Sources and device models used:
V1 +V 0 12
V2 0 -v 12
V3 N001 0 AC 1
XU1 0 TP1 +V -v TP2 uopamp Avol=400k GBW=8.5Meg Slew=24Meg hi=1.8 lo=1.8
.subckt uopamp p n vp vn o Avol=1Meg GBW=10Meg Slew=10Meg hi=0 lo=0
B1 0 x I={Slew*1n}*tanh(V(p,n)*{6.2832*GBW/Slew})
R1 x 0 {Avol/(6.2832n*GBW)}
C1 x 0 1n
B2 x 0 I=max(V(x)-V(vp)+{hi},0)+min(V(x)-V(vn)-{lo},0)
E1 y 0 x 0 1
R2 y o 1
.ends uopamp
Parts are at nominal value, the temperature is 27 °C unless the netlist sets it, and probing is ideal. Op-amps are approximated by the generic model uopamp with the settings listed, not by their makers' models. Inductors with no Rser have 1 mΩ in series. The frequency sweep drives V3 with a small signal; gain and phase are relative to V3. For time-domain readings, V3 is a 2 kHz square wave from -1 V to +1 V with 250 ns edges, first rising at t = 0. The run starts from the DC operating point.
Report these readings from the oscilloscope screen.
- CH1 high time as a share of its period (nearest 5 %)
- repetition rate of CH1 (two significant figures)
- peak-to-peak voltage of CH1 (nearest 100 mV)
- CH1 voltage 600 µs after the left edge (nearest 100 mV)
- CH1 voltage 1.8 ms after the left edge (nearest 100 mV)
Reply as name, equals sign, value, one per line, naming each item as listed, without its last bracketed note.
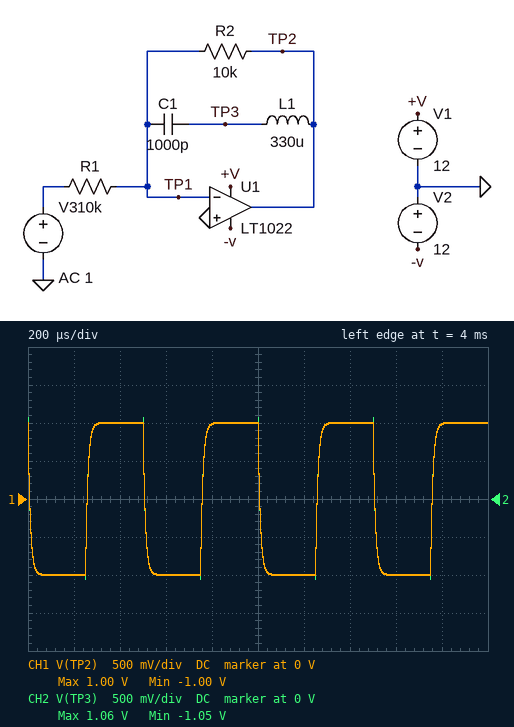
CH1 high time as a share of its period = 50 %
repetition rate of CH1 = 2.0 kHz
peak-to-peak voltage of CH1 = 2.0 V
CH1 voltage 600 µs after the left edge = -1.0 V
CH1 voltage 1.8 ms after the left edge = 1.0 V
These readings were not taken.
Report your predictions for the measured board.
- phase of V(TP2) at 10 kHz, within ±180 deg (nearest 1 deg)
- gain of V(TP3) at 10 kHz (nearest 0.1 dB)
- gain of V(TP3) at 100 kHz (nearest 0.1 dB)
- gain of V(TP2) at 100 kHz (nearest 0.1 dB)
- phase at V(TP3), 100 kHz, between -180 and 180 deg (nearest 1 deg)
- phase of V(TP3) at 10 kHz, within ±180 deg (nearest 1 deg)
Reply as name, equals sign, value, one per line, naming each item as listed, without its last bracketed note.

phase of V(TP2) at 10 kHz, within ±180 deg = 148 deg
gain of V(TP3) at 10 kHz = -1.4 dB
gain of V(TP3) at 100 kHz = -16.1 dB
gain of V(TP2) at 100 kHz = -17.3 dB
phase at V(TP3), 100 kHz, between -180 and 180 deg = 97 deg
phase of V(TP3) at 10 kHz, within ±180 deg = 148 deg
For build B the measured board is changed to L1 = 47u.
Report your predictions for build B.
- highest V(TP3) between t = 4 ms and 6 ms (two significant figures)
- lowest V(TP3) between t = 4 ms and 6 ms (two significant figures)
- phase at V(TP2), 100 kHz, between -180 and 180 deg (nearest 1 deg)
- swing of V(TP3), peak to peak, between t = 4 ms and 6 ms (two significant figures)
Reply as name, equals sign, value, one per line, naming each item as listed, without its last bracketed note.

highest V(TP3) between t = 4 ms and 6 ms = 1.0 V
lowest V(TP3) between t = 4 ms and 6 ms = -1.0 V
phase at V(TP2), 100 kHz, between -180 and 180 deg = 98 deg
swing of V(TP3), peak to peak, between t = 4 ms and 6 ms = 2.0 V
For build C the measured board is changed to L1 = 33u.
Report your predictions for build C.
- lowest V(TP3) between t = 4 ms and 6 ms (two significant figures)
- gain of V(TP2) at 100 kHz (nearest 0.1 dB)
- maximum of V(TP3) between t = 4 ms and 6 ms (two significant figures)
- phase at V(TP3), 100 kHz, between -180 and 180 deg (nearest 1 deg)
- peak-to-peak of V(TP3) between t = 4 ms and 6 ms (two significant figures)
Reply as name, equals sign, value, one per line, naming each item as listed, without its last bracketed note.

lowest V(TP3) between t = 4 ms and 6 ms = -1.0 V
gain of V(TP2) at 100 kHz = -16.2 dB
maximum of V(TP3) between t = 4 ms and 6 ms = 1.0 V
phase at V(TP3), 100 kHz, between -180 and 180 deg = 98 deg
peak-to-peak of V(TP3) between t = 4 ms and 6 ms = 2.0 V
